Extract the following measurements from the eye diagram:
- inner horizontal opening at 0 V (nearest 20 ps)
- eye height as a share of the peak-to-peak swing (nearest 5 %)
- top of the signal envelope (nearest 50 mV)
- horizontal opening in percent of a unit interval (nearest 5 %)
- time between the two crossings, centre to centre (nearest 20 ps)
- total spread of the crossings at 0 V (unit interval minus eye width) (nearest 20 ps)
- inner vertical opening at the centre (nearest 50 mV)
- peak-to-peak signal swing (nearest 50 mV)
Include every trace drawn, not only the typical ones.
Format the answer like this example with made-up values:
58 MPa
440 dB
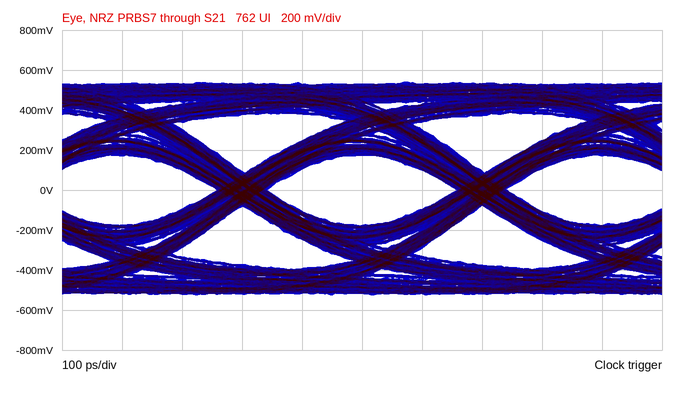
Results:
320 ps
35 %
550 mV
80 %
400 ps
80 ps
350 mV
1.05 V
